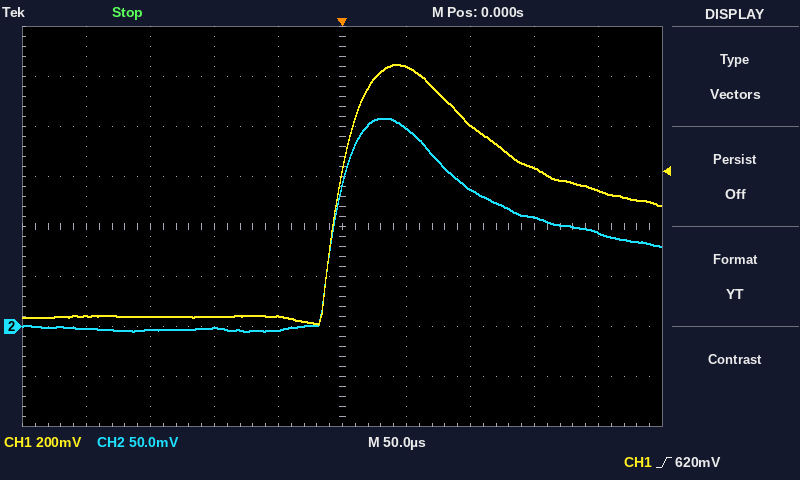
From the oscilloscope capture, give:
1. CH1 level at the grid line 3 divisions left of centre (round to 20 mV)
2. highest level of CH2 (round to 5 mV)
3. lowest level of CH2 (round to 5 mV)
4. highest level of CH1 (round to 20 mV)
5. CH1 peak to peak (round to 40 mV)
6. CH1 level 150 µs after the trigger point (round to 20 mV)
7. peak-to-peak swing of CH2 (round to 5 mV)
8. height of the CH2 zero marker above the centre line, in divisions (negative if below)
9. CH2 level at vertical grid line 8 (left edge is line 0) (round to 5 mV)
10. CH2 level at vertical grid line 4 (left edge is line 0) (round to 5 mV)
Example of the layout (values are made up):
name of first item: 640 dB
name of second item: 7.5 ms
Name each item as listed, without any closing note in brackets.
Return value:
CH1 level at the grid line 3 divisions left of centre: 40 mV
highest level of CH2: 210 mV
lowest level of CH2: -5 mV
highest level of CH1: 1.04 V
CH1 peak to peak: 1.04 V
CH1 level 150 µs after the trigger point: 640 mV
peak-to-peak swing of CH2: 215 mV
height of the CH2 zero marker above the centre line, in divisions: -2.0 div
CH2 level at vertical grid line 8 (left edge is line 0): 110 mV
CH2 level at vertical grid line 4 (left edge is line 0): -5 mV
